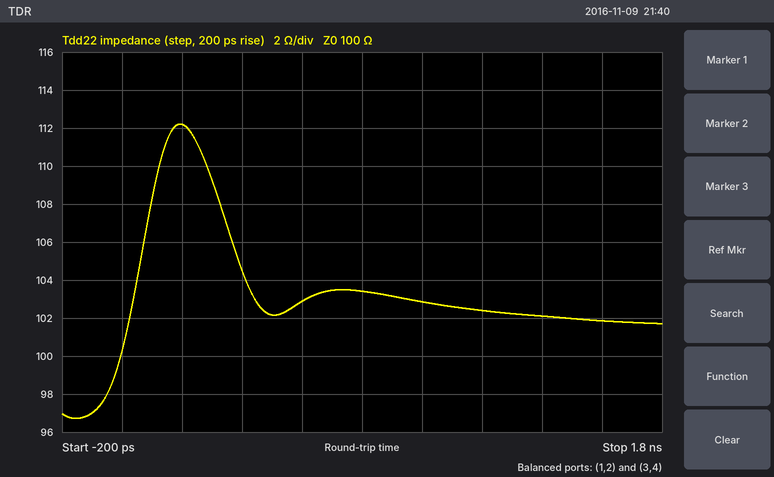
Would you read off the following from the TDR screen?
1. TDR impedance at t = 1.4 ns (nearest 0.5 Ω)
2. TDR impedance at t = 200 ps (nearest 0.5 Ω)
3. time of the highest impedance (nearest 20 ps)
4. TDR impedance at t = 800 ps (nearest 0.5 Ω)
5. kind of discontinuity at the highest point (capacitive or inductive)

102.0 Ω
112.0 Ω
200 ps
103.5 Ω
inductive
